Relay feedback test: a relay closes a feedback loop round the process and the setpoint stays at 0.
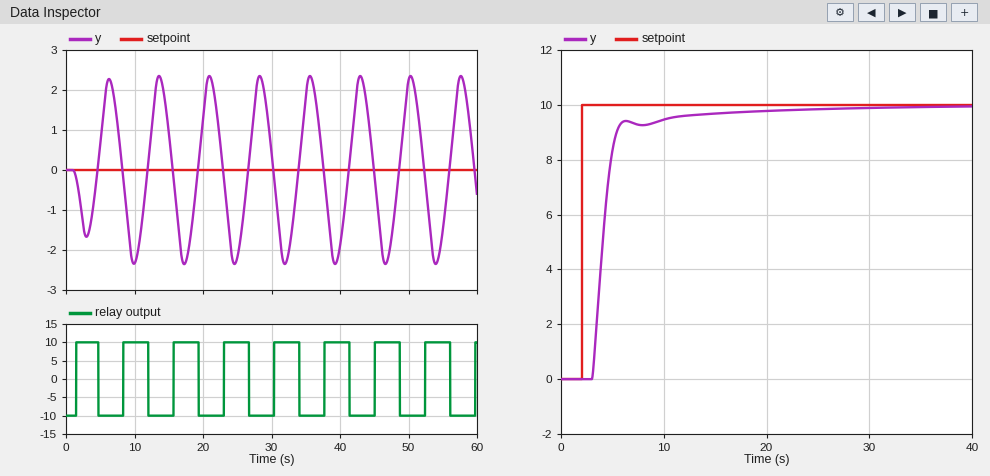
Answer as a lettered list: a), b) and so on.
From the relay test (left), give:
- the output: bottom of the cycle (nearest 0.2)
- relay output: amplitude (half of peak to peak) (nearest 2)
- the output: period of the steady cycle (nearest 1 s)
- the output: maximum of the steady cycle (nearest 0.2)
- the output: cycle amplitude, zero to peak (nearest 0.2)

a) -2.4
b) 10
c) 7 s
d) 2.4
e) 2.4
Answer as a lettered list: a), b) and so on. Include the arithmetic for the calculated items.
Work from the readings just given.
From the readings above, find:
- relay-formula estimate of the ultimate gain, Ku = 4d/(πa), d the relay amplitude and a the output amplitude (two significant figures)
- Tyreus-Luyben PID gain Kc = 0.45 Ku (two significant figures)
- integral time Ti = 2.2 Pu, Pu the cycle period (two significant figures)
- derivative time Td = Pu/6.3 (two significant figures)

a) 4 × 10 / (π × 2.4) = 5.3
b) 0.45 × 5.3 = 2.4
c) 2.2 × 7 = 15 s
d) 7 / 6.3 = 1.1 s
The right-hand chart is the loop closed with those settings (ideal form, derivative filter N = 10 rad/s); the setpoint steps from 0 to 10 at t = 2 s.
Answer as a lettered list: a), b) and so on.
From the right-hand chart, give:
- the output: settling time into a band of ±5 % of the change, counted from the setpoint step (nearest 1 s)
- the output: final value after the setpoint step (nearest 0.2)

a) 8 s
b) 10.0
